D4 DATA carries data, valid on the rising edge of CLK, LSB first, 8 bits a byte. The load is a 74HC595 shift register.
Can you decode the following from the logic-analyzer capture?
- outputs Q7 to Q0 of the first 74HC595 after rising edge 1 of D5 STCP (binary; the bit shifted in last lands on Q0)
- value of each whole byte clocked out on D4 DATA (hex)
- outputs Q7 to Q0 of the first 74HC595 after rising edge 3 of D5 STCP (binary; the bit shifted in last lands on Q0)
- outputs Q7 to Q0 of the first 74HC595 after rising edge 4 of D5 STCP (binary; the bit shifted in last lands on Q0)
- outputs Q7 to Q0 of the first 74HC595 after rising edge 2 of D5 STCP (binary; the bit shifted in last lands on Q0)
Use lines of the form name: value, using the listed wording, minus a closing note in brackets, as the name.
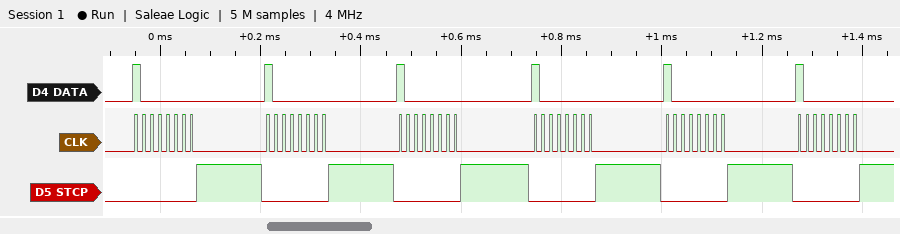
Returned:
outputs Q7 to Q0 of the first 74HC595 after rising edge 1 of D5 STCP: 10000000
value of each whole byte clocked out on D4 DATA: 0x01 0x01 0x01 0x01 0x01 0x01
outputs Q7 to Q0 of the first 74HC595 after rising edge 3 of D5 STCP: 10000000
outputs Q7 to Q0 of the first 74HC595 after rising edge 4 of D5 STCP: 10000000
outputs Q7 to Q0 of the first 74HC595 after rising edge 2 of D5 STCP: 10000000
